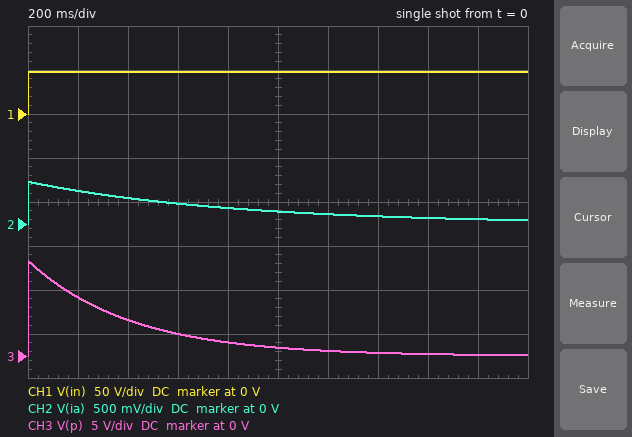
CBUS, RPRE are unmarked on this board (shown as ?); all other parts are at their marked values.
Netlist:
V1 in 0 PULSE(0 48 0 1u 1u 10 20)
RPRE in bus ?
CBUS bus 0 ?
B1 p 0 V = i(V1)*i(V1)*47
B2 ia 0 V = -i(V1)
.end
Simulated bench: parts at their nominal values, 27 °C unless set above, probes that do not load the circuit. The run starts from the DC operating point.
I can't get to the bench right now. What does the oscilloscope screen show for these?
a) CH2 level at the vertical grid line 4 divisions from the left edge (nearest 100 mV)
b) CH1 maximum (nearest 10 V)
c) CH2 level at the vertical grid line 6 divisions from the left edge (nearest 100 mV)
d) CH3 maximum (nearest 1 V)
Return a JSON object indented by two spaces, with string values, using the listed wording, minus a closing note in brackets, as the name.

{
  "CH2 level at the vertical grid line 4 divisions from the left edge": "200 mV",
  "CH1 maximum": "50 V",
  "CH2 level at the vertical grid line 6 divisions from the left edge": "100 mV",
  "CH3 maximum": "11 V"
}
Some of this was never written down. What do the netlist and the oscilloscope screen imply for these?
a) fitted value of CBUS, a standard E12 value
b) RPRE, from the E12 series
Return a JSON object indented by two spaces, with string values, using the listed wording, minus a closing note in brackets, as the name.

{
  "fitted value of CBUS, a standard E12 value": "8.2 mF",
  "RPRE, from the E12 series": "100 Ω"
}
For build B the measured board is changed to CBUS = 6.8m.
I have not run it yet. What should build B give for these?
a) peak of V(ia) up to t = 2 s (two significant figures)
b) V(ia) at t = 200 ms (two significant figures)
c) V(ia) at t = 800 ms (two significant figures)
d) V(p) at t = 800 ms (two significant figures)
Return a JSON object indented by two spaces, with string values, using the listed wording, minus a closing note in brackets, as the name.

{
  "peak of V(ia) up to t = 2 s": "480 mV",
  "V(ia) at t = 200 ms": "360 mV",
  "V(ia) at t = 800 ms": "150 mV",
  "V(p) at t = 800 ms": "1.0 V"
}
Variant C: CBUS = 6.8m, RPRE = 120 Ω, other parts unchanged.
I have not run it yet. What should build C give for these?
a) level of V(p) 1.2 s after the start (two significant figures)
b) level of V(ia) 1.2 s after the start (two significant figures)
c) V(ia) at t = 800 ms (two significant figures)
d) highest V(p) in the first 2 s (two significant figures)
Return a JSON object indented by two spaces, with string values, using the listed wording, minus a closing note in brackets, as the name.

{
  "level of V(p) 1.2 s after the start": "400 mV",
  "level of V(ia) 1.2 s after the start": "92 mV",
  "V(ia) at t = 800 ms": "150 mV",
  "highest V(p) in the first 2 s": "7.5 V"
}
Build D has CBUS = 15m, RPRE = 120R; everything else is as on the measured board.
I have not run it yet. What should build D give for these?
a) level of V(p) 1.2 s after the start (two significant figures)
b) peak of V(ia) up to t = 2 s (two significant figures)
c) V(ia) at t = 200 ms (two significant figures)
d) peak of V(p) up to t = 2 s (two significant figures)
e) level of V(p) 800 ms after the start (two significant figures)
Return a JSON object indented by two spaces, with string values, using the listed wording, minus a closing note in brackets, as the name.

{
  "level of V(p) 1.2 s after the start": "2.0 V",
  "peak of V(ia) up to t = 2 s": "400 mV",
  "V(ia) at t = 200 ms": "360 mV",
  "peak of V(p) up to t = 2 s": "7.5 V",
  "level of V(p) 800 ms after the start": "3.1 V"
}
